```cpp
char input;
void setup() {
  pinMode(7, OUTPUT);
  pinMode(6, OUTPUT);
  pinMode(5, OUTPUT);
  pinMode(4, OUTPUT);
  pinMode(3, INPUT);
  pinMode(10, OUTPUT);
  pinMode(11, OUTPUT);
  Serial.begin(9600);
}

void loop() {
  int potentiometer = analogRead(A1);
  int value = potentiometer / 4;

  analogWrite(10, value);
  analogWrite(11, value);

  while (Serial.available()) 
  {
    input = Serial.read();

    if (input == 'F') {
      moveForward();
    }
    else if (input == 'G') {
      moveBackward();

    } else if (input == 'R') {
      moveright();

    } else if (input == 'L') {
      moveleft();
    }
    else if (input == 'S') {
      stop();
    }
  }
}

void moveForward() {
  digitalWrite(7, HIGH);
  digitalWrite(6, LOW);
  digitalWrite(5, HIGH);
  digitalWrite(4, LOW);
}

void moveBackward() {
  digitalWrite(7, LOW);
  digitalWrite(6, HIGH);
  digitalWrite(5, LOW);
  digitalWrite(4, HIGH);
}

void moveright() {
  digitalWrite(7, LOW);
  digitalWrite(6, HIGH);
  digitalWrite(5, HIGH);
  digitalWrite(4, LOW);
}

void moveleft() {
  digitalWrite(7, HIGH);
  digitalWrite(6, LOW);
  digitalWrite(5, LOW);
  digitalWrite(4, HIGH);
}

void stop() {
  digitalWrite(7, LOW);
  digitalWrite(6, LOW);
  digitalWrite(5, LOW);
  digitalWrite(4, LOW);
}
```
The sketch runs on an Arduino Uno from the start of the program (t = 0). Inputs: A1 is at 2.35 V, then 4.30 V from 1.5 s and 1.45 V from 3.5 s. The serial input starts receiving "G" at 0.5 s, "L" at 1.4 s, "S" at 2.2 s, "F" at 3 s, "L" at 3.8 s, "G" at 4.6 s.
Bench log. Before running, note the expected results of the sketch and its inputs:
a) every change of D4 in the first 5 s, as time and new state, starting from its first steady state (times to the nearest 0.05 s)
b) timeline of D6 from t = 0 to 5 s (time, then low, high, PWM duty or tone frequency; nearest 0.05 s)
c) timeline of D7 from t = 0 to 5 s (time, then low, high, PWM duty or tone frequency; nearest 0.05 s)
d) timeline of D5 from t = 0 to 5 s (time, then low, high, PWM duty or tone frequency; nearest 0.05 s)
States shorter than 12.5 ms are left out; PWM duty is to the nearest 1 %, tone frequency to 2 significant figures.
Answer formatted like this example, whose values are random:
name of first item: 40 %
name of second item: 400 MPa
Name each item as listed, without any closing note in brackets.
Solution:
every change of D4 in the first 5 s, as time and new state, starting from its first steady state: 0 s low; 0.5 s high; 2.2 s low; 3.8 s high
timeline of D6 from t = 0 to 5 s: 0 s low; 0.5 s high; 1.4 s low; 4.6 s high
timeline of D7 from t = 0 to 5 s: 0 s low; 1.4 s high; 2.2 s low; 3 s high; 4.6 s low
timeline of D5 from t = 0 to 5 s: 0 s low; 3 s high; 3.8 s low
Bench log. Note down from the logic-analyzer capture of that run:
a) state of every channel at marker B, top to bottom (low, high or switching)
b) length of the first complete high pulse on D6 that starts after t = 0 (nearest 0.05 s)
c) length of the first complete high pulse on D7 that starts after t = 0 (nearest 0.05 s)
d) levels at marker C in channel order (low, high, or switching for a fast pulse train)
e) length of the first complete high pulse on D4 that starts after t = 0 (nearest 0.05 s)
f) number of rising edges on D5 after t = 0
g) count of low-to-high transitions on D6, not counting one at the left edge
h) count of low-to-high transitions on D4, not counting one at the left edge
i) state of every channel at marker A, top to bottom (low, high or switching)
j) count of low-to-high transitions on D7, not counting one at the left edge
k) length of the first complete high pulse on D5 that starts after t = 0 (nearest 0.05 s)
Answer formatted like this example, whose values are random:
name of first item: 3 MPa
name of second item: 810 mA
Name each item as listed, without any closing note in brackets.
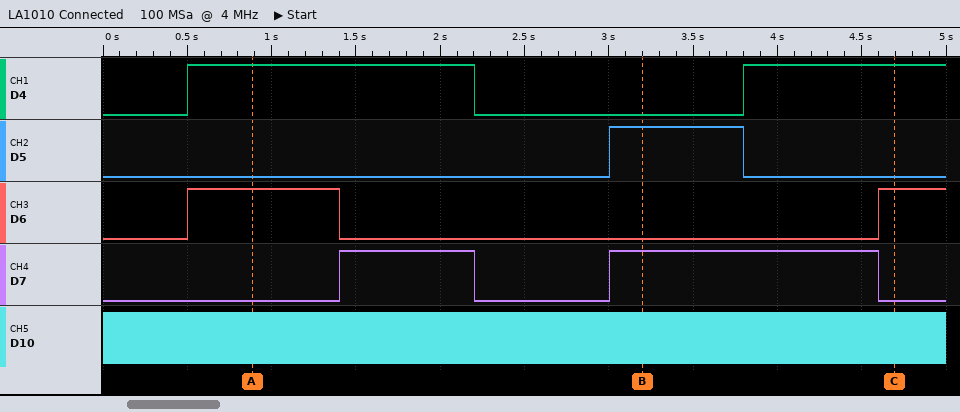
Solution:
state of every channel at marker B, top to bottom: D4 low, D5 high, D6 low, D7 high, D10 switching
length of the first complete high pulse on D6 that starts after t = 0: 0.90 s
length of the first complete high pulse on D7 that starts after t = 0: 0.80 s
levels at marker C in channel order: D4 high, D5 low, D6 high, D7 low, D10 switching
length of the first complete high pulse on D4 that starts after t = 0: 1.70 s
number of rising edges on D5 after t = 0: 1
count of low-to-high transitions on D6, not counting one at the left edge: 2
count of low-to-high transitions on D4, not counting one at the left edge: 2
state of every channel at marker A, top to bottom: D4 high, D5 low, D6 high, D7 low, D10 switching
count of low-to-high transitions on D7, not counting one at the left edge: 2
length of the first complete high pulse on D5 that starts after t = 0: 0.80 s
